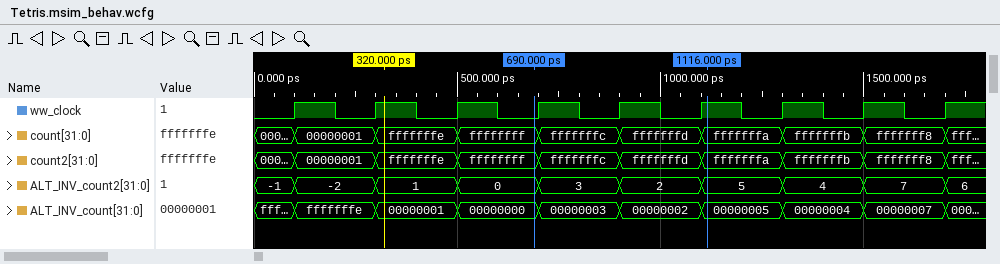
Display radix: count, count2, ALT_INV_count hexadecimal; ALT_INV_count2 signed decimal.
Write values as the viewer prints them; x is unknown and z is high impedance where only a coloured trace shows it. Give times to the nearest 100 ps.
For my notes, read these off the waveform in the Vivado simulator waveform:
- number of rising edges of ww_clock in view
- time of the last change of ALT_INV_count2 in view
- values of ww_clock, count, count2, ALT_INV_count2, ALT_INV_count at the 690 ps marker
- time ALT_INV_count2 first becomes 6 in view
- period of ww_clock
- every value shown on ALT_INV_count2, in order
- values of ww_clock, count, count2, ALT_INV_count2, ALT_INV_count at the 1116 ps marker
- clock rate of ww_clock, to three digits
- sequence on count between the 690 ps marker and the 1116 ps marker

9
1700 ps
ww_clock=0, count=ffffffff, count2=ffffffff, ALT_INV_count2=0, ALT_INV_count=00000000
1700 ps
200 ps
-1, -2, 1, 0, 3, 2, 5, 4, 7, 6
ww_clock=1, count=fffffffa, count2=fffffffa, ALT_INV_count2=5, ALT_INV_count=00000005
5.00 GHz
ffffffff, fffffffc, fffffffd, fffffffa
